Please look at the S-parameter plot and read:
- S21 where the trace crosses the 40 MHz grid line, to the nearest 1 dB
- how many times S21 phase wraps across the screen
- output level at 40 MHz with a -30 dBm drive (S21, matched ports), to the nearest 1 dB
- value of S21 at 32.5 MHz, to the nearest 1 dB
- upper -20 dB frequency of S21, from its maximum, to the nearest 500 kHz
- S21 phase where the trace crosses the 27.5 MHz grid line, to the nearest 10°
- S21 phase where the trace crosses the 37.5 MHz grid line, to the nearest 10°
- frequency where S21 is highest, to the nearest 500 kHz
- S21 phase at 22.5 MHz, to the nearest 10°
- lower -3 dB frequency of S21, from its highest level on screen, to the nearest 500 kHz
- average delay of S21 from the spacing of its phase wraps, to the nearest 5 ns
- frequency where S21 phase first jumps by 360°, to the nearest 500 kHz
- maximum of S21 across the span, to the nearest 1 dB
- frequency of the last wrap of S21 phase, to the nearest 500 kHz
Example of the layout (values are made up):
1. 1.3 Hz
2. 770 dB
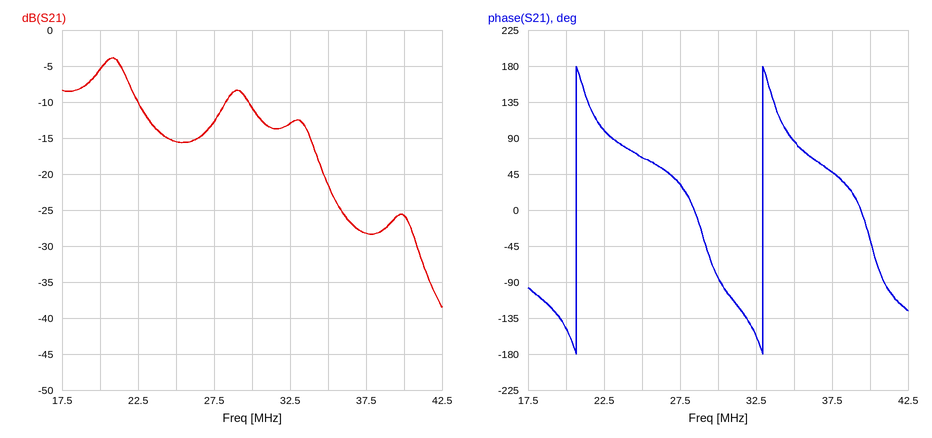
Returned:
1. -26 dB
2. 2
3. -56 dBm
4. -13 dB
5. 35.5 MHz
6. 30°
7. 50°
8. 21.0 MHz
9. 100°
10. 19.5 MHz
11. 80 ns
12. 20.5 MHz
13. -4 dB
14. 33.0 MHz
